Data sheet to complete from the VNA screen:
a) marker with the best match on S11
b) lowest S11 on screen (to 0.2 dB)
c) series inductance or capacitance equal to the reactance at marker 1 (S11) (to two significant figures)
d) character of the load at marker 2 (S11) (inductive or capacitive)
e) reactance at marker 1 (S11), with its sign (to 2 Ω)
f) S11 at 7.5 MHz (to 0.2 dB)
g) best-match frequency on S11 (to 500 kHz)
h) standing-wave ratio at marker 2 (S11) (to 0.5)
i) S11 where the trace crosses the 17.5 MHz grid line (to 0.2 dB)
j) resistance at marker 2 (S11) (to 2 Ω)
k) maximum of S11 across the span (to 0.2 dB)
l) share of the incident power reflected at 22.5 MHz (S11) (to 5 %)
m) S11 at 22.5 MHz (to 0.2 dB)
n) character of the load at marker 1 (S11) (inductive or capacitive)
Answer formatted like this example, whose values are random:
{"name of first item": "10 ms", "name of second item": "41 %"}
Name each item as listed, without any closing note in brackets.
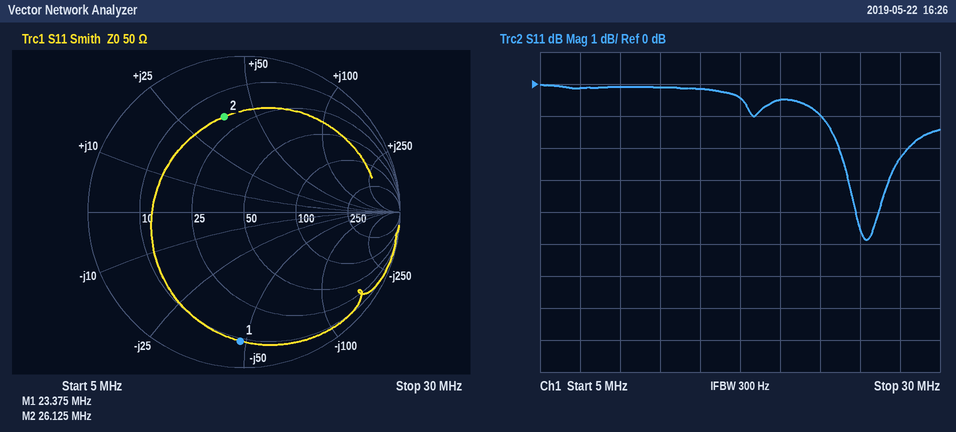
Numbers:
{"marker with the best match on S11": "marker 2", "lowest S11 on screen": "-4.8 dB", "series inductance or capacitance equal to the reactance at marker 1 (S11)": "140 pF", "character of the load at marker 2 (S11)": "inductive", "reactance at marker 1 (S11), with its sign": "-48 Ω", "S11 at 7.5 MHz": "-0.2 dB", "best-match frequency on S11": "25.5 MHz", "standing-wave ratio at marker 2 (S11)": "4.5", "S11 where the trace crosses the 17.5 MHz grid line": "-0.4 dB", "resistance at marker 2 (S11)": "18 Ω", "maximum of S11 across the span": "0.0 dB", "share of the incident power reflected at 22.5 MHz (S11)": "80 %", "S11 at 22.5 MHz": "-1.0 dB", "character of the load at marker 1 (S11)": "capacitive"}
